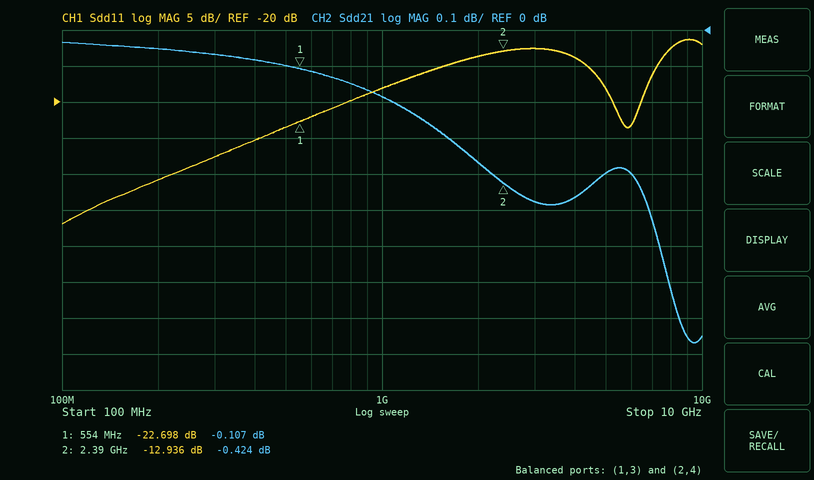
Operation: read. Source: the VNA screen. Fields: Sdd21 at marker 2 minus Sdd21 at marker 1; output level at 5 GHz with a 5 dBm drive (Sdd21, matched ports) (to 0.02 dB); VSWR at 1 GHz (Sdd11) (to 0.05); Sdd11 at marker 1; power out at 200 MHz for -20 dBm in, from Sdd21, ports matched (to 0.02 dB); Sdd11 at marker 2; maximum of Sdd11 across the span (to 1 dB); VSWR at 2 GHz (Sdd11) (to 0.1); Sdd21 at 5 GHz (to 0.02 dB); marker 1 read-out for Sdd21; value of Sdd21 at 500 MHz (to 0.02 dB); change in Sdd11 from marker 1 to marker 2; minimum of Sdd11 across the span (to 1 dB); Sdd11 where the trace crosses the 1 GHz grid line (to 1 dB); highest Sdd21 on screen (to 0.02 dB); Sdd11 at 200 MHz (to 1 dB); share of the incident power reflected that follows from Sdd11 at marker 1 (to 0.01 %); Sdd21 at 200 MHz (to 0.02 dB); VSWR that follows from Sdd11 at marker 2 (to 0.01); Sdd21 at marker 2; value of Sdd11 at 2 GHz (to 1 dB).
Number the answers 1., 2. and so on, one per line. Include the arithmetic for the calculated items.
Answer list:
1. -0.424 − (-0.107) = -0.317 dB
2. 5 dBm + (-0.40 dB) = 4.60 dBm
3. |Γ| = 10^(-18/20) = 0.1259; VSWR = (1 + 0.1259)/(1 − 0.1259) ≈ 1.29, so 1.30 to the nearest 0.05
4. -22.698 dB
5. -20 dBm + (-0.06 dB) = -20.06 dBm
6. -12.936 dB
7. -11 dB
8. |Γ| = 10^(-14/20) = 0.1995; VSWR = (1 + 0.1995)/(1 − 0.1995) ≈ 1.5
9. -0.40 dB
10. -0.107 dB
11. -0.10 dB
12. -12.936 − (-22.698) = 9.762 dB
13. -37 dB
14. -18 dB
15. -0.04 dB
16. -31 dB
17. 10^(-22.698/10) ≈ 0.54 %
18. -0.06 dB
19. (1 + 0.2255)/(1 − 0.2255) ≈ 1.58
20. -0.424 dB
21. -14 dB
